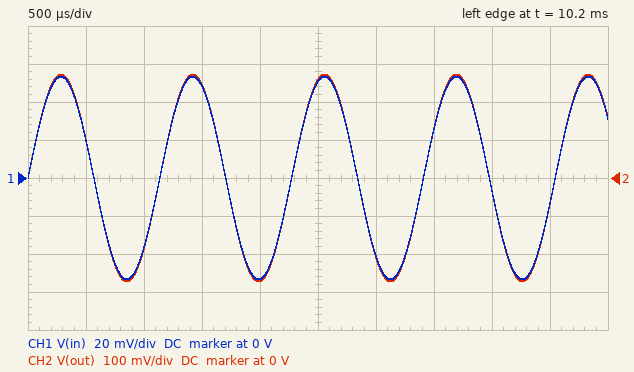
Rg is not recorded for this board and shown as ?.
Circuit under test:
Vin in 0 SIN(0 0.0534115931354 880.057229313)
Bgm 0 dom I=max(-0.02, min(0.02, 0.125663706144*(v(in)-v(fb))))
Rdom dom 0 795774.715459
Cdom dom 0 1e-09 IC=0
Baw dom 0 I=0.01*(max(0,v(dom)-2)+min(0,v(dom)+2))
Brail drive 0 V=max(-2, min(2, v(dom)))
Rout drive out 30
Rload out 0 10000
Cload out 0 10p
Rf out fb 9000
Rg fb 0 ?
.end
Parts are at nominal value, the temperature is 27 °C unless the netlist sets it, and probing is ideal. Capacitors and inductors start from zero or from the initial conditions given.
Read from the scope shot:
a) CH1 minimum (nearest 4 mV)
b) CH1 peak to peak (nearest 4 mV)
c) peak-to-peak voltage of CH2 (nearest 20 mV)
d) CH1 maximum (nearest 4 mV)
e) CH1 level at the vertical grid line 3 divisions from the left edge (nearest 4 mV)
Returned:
-52 mV
108 mV
540 mV
52 mV
48 mV
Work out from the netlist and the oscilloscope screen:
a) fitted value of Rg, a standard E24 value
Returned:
2.2 kΩ
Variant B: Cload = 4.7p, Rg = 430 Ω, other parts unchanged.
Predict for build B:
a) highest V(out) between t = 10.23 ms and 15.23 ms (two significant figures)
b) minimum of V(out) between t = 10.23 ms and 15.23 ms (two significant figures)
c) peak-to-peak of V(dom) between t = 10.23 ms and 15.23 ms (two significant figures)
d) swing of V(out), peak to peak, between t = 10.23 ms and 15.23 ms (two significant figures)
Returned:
1.2 V
-1.2 V
2.4 V
2.3 V
